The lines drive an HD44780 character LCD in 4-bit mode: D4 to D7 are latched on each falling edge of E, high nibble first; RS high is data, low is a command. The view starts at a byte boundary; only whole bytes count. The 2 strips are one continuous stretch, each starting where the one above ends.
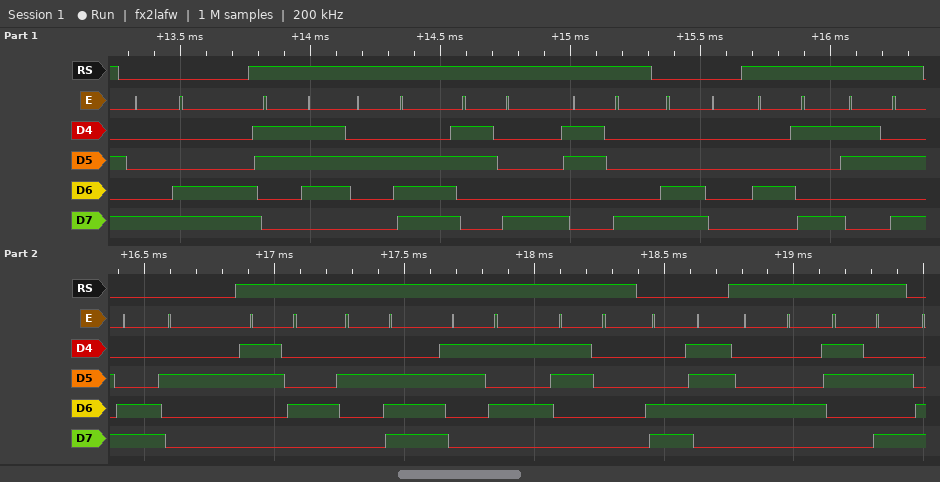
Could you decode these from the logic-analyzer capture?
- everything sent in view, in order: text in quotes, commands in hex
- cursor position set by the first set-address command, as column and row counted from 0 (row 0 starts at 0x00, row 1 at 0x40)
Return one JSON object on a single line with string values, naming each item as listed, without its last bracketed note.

{"everything sent in view, in order: text in quotes, commands in hex": "0x8C \"7.88\" 0xC0 \"I:\" 0xC2 \"4.50\" 0xC7 \"D:\"", "cursor position set by the first set-address command, as column and row counted from 0": "column 12, row 0"}
